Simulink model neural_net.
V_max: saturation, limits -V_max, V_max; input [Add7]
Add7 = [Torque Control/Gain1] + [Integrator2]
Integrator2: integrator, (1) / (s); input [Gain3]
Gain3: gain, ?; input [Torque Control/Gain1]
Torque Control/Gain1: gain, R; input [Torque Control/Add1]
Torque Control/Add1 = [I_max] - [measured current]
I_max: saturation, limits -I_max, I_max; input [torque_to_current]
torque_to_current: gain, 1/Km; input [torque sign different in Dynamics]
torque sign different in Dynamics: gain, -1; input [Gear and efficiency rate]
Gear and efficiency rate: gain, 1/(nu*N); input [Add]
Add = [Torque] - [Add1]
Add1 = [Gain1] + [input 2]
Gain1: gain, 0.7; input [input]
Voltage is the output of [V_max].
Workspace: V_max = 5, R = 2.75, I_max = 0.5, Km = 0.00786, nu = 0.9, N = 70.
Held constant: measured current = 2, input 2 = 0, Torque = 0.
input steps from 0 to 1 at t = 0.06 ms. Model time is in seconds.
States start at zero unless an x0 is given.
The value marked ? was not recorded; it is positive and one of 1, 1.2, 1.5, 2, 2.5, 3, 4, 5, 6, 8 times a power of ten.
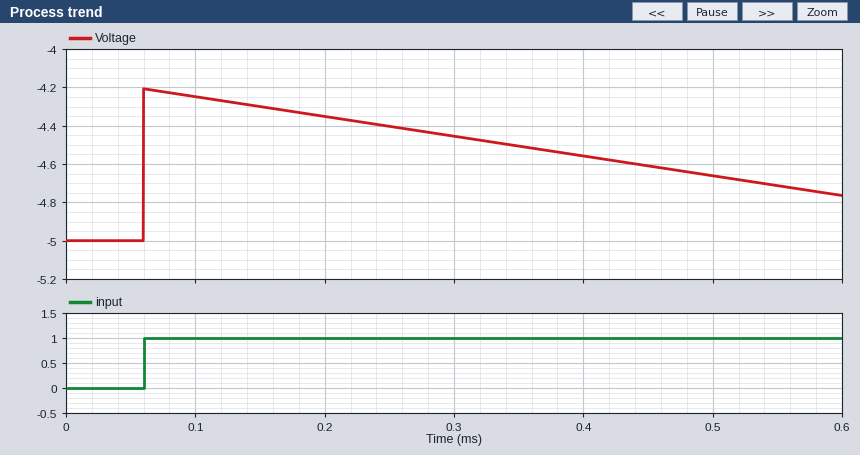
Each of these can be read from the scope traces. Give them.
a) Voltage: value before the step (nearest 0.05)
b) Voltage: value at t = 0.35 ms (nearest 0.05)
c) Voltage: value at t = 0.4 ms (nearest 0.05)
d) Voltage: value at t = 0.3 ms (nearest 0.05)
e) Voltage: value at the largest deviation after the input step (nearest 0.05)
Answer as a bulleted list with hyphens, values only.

- -5.00
- -4.50
- -4.55
- -4.45
- -4.20
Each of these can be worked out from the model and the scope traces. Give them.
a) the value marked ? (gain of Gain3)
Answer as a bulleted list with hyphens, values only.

- 250
